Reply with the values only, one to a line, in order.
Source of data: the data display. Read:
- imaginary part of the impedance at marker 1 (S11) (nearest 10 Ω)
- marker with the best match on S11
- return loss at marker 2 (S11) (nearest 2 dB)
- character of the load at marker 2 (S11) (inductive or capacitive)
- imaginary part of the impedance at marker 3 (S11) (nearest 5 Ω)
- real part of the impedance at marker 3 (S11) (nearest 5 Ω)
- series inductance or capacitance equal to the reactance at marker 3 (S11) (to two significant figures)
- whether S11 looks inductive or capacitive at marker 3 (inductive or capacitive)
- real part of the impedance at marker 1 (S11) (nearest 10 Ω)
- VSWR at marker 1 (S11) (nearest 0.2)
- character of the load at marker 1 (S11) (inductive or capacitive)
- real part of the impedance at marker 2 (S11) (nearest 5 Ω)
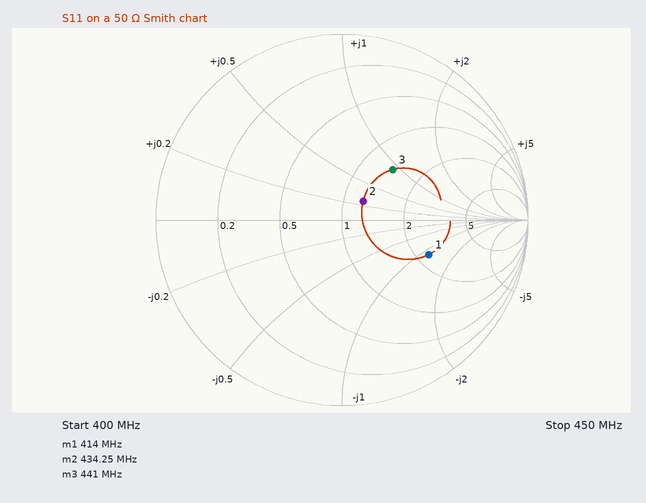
-60 Ω
marker 2
16 dB
inductive
+45 Ω
70 Ω
16 nH
inductive
120 Ω
3.0
capacitive
60 Ω
